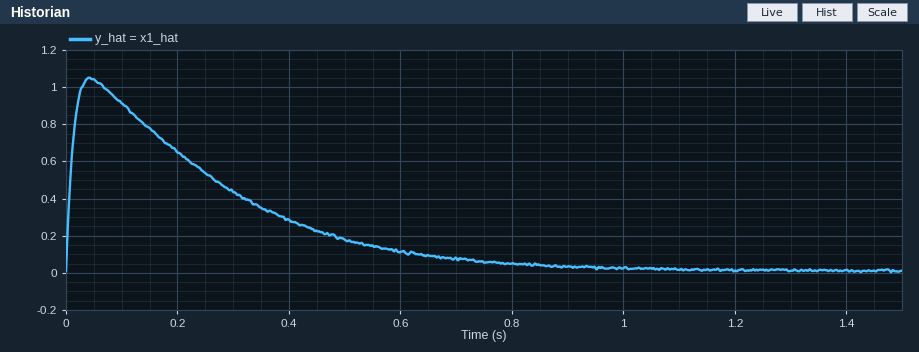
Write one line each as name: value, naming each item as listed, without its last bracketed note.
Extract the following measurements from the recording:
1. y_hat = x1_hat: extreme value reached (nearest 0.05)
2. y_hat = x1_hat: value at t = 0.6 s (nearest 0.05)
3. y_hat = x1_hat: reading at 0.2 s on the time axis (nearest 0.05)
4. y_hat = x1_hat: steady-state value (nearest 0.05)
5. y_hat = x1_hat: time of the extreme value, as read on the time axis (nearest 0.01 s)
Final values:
y_hat = x1_hat: extreme value reached: 1.05
y_hat = x1_hat: value at t = 0.6 s: 0.10
y_hat = x1_hat: reading at 0.2 s on the time axis: 0.65
y_hat = x1_hat: steady-state value: 0.00
y_hat = x1_hat: time of the extreme value, as read on the time axis: 0.04 s
